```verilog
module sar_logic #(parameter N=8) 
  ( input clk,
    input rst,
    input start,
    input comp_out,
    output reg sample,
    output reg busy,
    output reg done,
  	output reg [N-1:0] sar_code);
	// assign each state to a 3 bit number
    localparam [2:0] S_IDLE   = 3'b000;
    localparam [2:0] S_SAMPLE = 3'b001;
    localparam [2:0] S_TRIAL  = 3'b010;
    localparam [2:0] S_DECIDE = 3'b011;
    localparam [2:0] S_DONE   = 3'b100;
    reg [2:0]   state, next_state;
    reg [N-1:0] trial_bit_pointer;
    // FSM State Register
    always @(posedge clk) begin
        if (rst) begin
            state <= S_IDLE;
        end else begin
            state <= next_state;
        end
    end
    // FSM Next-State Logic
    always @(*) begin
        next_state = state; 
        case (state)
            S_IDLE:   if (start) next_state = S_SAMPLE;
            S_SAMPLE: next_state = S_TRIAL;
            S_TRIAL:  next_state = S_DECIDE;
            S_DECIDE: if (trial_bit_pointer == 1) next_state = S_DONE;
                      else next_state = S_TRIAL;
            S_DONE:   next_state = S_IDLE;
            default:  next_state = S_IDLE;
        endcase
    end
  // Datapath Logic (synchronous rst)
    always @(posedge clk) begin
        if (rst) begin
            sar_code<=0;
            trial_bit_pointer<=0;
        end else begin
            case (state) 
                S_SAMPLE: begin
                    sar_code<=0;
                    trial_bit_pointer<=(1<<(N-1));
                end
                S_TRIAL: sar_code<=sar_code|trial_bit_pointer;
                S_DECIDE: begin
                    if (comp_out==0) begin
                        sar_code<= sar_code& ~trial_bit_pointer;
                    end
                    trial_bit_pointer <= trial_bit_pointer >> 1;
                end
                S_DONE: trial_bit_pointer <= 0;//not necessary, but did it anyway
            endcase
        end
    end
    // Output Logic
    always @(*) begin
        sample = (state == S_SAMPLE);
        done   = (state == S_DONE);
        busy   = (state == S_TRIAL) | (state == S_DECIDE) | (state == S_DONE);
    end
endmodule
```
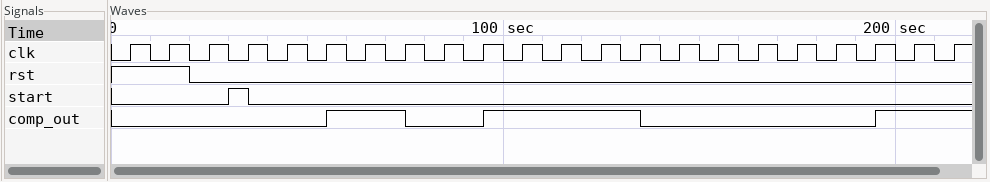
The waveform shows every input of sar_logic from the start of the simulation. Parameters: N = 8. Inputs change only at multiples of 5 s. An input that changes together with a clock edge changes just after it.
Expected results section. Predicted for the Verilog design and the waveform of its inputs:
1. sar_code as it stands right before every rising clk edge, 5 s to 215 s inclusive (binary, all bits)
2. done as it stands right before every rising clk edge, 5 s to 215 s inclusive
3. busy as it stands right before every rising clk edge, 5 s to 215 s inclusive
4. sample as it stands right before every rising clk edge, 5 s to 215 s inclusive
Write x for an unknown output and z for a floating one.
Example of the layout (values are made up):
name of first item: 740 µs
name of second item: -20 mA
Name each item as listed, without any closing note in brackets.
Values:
sar_code as it stands right before every rising clk edge, 5 s to 215 s inclusive: x, 00000000, 00000000, 00000000, 00000000, 00000000, 10000000, 10000000, 11000000, 10000000, 10100000, 10100000, 10110000, 10110000, 10111000, 10110000, 10110100, 10110000, 10110010, 10110000, 10110001, 10110001
done as it stands right before every rising clk edge, 5 s to 215 s inclusive: x 0 0 0 0 0 0 0 0 0 0 0 0 0 0 0 0 0 0 0 0 1
busy as it stands right before every rising clk edge, 5 s to 215 s inclusive: x 0 0 0 0 1 1 1 1 1 1 1 1 1 1 1 1 1 1 1 1 1
sample as it stands right before every rising clk edge, 5 s to 215 s inclusive: x 0 0 0 1 0 0 0 0 0 0 0 0 0 0 0 0 0 0 0 0 0
